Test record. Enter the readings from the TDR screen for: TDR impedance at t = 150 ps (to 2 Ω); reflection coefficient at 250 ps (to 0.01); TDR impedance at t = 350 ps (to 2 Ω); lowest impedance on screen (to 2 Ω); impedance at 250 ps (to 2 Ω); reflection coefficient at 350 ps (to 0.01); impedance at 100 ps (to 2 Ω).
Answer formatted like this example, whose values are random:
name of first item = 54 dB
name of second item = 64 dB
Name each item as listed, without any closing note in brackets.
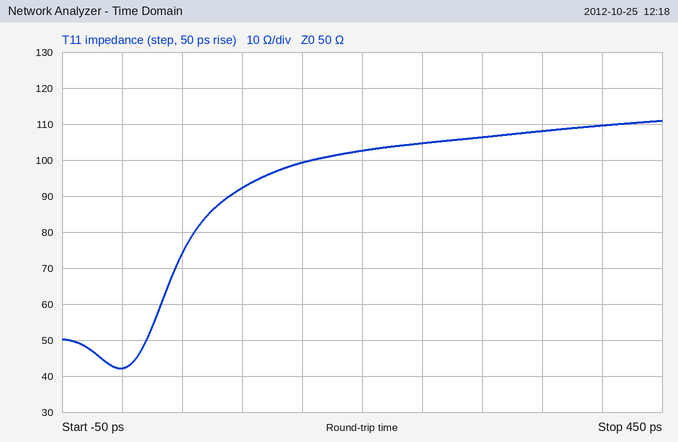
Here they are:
TDR impedance at t = 150 ps = 100 Ω
reflection coefficient at 250 ps = +0.35
TDR impedance at t = 350 ps = 108 Ω
lowest impedance on screen = 42 Ω
impedance at 250 ps = 104 Ω
reflection coefficient at 350 ps = +0.37
impedance at 100 ps = 92 Ω
